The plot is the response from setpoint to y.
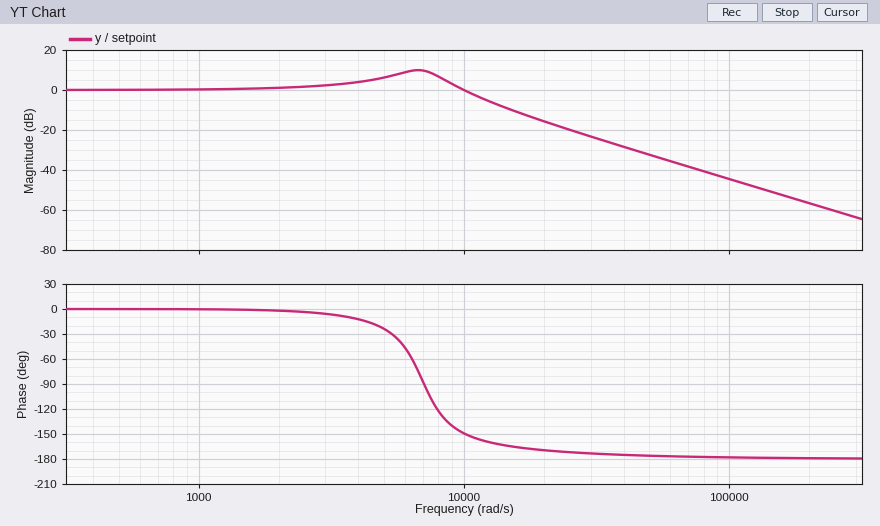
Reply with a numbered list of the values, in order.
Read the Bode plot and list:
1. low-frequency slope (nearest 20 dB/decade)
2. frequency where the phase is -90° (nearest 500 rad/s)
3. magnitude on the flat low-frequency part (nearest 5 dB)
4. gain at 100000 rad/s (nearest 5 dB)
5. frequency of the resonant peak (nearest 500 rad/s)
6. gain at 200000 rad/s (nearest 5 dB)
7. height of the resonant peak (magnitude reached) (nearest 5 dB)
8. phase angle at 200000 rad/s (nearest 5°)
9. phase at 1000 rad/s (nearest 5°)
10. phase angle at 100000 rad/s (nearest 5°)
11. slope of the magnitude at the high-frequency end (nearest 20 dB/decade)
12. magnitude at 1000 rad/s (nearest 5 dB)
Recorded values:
1. 0 dB/decade
2. 7000 rad/s
3. 0 dB
4. -45 dB
5. 6500 rad/s
6. -55 dB
7. 10 dB
8. -180°
9. 0°
10. -180°
11. -40 dB/decade
12. 0 dB
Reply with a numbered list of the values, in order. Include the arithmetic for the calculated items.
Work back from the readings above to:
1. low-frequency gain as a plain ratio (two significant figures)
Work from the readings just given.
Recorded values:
1. 10^(0 / 20) = 1.0
